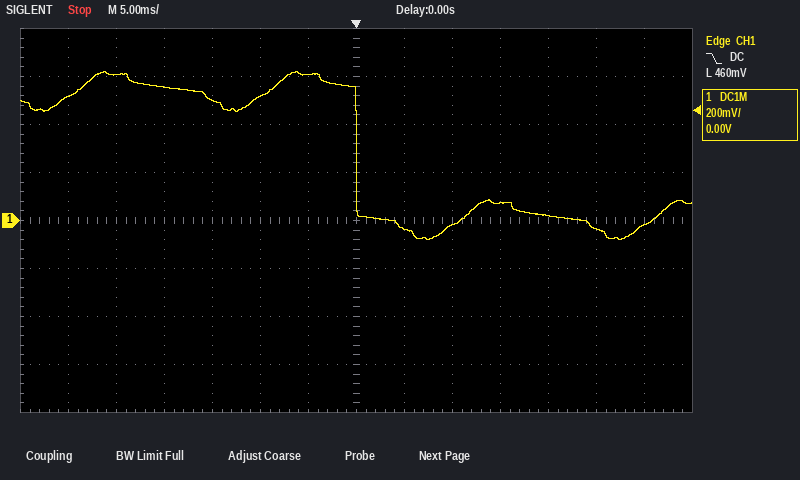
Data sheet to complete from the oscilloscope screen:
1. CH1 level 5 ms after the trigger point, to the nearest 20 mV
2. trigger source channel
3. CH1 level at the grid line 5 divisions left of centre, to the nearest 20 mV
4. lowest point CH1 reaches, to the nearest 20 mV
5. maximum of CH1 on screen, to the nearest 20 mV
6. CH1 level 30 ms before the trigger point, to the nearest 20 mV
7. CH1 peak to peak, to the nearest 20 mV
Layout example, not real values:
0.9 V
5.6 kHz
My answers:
-40 mV
CH1
600 mV
-80 mV
620 mV
520 mV
700 mV
